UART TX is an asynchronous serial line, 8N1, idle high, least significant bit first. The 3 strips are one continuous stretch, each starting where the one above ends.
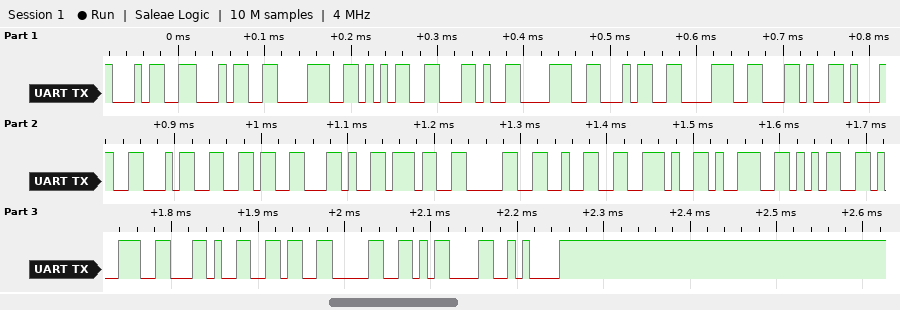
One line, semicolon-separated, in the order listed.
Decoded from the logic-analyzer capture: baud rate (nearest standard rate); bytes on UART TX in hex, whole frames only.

115200 baud; 34 34 38 35 2C 38 34 38 2C 31 34 36 2C 37 30 32 2E 39 35 39 2C 36 30 0D 0A
